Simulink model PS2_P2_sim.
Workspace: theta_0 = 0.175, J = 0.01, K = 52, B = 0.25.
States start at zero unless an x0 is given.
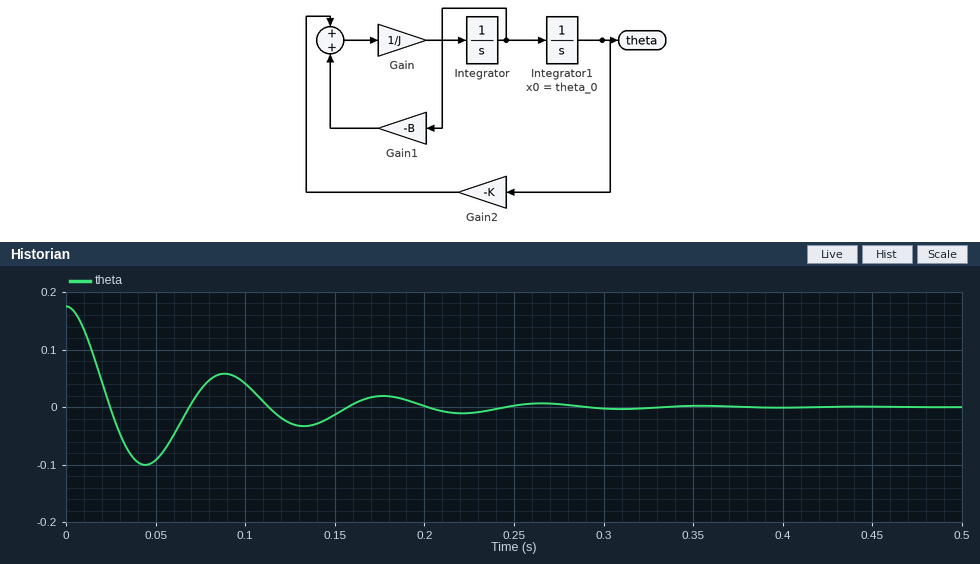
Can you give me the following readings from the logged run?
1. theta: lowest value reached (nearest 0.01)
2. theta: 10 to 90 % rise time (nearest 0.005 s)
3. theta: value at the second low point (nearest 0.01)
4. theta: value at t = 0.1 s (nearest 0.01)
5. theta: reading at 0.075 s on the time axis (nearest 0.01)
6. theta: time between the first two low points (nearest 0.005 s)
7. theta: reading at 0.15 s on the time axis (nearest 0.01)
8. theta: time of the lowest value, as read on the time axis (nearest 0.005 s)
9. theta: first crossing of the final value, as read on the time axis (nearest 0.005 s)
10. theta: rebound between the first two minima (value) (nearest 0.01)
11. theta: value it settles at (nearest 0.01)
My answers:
-0.10
0.015 s
-0.03
0.04
0.03
0.090 s
-0.01
0.045 s
0.025 s
0.06
0.00
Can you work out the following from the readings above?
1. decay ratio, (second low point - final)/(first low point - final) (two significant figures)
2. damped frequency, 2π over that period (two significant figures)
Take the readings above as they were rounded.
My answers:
0.30
70 rad/s
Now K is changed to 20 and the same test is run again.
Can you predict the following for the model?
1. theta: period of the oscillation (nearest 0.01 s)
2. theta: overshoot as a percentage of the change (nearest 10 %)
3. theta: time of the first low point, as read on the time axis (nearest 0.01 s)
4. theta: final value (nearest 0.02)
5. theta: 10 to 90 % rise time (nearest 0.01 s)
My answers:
0.15 s
40 %
0.07 s
0.00
0.03 s
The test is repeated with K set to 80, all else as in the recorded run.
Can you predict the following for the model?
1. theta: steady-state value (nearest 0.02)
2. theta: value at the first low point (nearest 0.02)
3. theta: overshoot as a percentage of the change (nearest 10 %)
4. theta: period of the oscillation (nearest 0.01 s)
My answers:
0.00
-0.12
60 %
0.07 s
